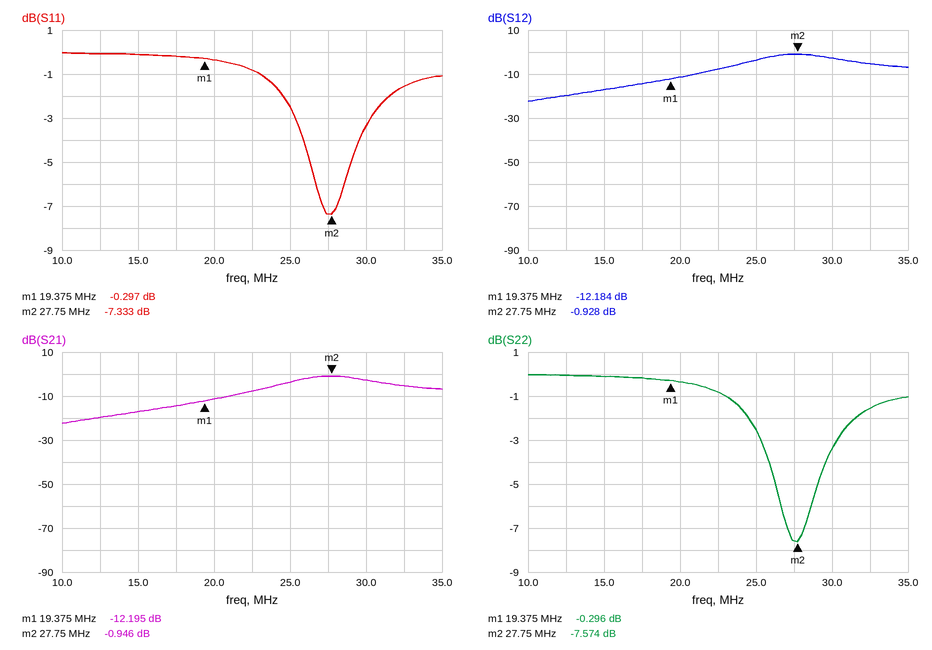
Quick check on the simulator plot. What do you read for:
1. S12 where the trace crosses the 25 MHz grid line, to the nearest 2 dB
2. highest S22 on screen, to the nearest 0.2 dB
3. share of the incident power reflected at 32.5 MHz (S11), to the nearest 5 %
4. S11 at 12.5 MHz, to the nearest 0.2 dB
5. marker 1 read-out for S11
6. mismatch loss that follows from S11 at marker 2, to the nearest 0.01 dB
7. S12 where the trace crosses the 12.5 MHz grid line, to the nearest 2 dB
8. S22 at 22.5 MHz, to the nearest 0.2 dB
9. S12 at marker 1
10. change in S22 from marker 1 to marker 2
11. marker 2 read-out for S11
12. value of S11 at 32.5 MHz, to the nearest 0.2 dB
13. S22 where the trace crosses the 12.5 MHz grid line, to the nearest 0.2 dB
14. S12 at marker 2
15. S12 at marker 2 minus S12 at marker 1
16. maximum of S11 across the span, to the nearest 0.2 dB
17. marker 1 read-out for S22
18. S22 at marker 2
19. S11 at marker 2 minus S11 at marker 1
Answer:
-4 dB
0.0 dB
70 %
0.0 dB
-0.297 dB
0.89 dB
-20 dB
-0.8 dB
-12.184 dB
-7.278 dB
-7.333 dB
-1.6 dB
0.0 dB
-0.928 dB
11.256 dB
0.0 dB
-0.296 dB
-7.574 dB
-7.036 dB
